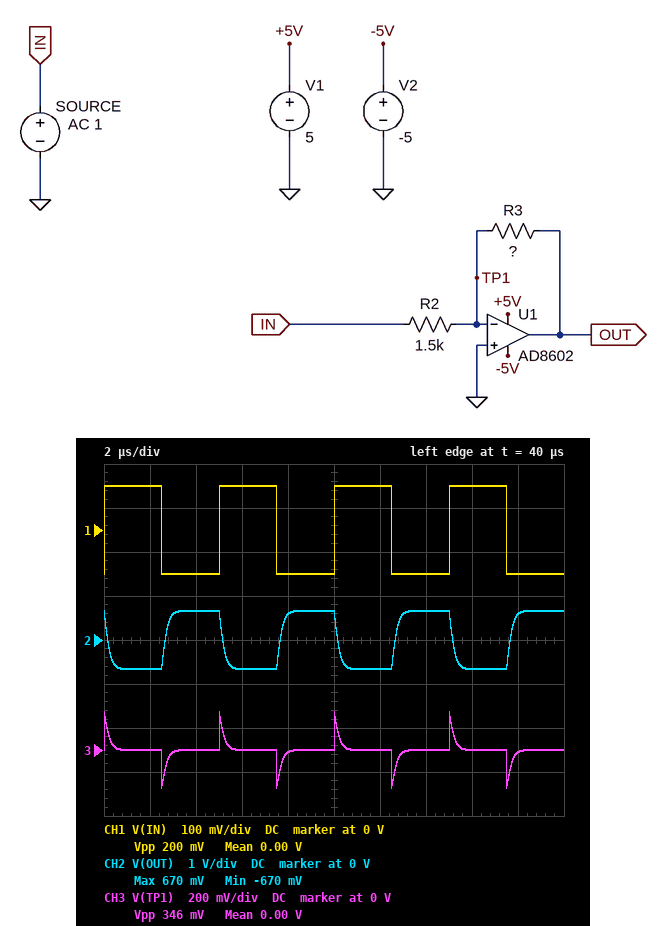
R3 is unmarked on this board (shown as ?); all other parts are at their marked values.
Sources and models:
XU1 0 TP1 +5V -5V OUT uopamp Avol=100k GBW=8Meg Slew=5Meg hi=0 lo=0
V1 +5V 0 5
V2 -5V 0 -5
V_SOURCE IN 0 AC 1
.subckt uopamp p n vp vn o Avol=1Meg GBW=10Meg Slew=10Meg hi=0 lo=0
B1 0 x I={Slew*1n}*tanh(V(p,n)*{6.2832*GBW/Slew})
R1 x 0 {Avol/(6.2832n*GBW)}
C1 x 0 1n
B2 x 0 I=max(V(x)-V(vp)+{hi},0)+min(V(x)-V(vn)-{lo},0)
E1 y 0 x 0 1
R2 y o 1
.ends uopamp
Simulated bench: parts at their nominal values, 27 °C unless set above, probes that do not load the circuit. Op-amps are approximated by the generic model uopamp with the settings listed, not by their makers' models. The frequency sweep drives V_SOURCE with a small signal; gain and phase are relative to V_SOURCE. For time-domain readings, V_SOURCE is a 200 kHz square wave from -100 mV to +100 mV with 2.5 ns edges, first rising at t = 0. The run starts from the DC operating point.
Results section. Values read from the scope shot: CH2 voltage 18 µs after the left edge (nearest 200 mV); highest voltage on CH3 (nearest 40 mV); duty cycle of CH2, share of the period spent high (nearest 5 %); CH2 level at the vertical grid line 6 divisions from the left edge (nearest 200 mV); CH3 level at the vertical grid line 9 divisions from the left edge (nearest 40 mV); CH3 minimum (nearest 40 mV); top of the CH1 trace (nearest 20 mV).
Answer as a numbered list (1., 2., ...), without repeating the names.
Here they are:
1. 600 mV
2. 160 mV
3. 50 %
4. -600 mV
5. 0 V
6. -160 mV
7. 100 mV
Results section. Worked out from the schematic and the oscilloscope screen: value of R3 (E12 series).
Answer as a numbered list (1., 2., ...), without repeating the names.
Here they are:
1. 10 kΩ
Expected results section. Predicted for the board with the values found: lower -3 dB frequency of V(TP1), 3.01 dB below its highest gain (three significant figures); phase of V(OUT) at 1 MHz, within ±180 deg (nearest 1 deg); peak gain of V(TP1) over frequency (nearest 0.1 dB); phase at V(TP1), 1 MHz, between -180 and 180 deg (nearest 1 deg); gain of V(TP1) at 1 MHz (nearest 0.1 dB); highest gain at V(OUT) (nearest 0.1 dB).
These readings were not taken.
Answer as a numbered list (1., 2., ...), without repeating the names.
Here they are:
1. 1.04 MHz
2. 136 deg
3. -1.2 dB
4. 46 deg
5. -4.4 dB
6. 16.5 dB
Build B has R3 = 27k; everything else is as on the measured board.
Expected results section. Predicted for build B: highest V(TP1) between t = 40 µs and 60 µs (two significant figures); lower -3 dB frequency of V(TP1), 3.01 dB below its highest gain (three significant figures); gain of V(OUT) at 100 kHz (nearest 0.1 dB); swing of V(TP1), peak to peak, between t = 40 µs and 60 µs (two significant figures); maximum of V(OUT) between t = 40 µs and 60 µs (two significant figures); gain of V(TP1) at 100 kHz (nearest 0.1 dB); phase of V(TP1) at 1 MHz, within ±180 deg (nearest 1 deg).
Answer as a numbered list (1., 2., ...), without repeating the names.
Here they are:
1. 190 mV
2. 421 kHz
3. 24.9 dB
4. 380 mV
5. 1.8 V
6. -13.2 dB
7. 23 deg
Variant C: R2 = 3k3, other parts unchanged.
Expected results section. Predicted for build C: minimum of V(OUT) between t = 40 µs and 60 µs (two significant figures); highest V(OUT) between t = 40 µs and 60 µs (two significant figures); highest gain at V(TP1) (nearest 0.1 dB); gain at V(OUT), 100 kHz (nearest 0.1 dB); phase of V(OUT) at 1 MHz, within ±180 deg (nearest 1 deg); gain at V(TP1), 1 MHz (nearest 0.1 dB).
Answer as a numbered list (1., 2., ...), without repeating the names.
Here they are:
1. -300 mV
2. 300 mV
3. -2.5 dB
4. 9.6 dB
5. 153 deg
6. -9.4 dB
